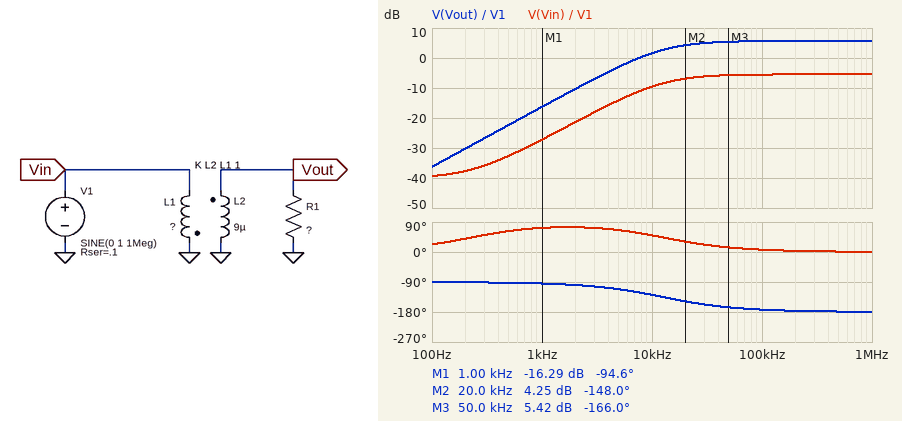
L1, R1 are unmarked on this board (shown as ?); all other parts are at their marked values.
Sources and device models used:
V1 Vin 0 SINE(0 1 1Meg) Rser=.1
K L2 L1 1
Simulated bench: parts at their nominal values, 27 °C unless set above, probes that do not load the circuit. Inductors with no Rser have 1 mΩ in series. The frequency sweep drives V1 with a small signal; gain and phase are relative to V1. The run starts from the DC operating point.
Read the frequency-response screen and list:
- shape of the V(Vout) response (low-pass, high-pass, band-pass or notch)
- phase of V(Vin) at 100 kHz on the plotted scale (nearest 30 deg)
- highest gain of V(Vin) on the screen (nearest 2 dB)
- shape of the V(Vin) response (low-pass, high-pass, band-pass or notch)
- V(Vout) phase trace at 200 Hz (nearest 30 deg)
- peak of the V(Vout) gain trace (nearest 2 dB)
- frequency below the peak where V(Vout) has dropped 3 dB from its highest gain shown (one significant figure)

high-pass
0 deg
-6 dB
high-pass
-90 deg
6 dB
10 kHz
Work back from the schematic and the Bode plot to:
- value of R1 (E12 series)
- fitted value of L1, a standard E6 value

1.5 Ω
680 nH
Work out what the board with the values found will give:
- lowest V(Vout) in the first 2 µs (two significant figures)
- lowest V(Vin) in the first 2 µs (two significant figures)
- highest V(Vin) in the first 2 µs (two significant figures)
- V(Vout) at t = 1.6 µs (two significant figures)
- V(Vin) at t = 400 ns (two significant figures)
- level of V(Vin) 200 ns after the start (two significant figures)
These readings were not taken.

-1.9 V
-540 mV
530 mV
1.2 V
300 mV
500 mV
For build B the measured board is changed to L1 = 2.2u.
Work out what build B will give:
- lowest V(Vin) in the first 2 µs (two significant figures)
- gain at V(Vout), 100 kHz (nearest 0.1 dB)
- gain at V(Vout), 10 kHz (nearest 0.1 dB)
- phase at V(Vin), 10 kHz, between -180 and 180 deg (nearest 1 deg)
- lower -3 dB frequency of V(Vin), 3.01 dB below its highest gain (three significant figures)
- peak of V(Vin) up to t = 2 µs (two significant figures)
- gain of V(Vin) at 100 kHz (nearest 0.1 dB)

-790 mV
4.0 dB
2.8 dB
29 deg
5.73 kHz
780 mV
-2.1 dB
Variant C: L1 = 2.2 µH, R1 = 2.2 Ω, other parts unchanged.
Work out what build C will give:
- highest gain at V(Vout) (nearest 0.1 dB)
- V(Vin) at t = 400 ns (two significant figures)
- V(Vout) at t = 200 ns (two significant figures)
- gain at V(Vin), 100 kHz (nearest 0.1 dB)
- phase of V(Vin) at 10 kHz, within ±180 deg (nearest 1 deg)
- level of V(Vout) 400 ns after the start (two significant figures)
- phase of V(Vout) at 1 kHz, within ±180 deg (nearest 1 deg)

4.6 dB
490 mV
-1.6 V
-1.5 dB
31 deg
-980 mV
-99 deg
